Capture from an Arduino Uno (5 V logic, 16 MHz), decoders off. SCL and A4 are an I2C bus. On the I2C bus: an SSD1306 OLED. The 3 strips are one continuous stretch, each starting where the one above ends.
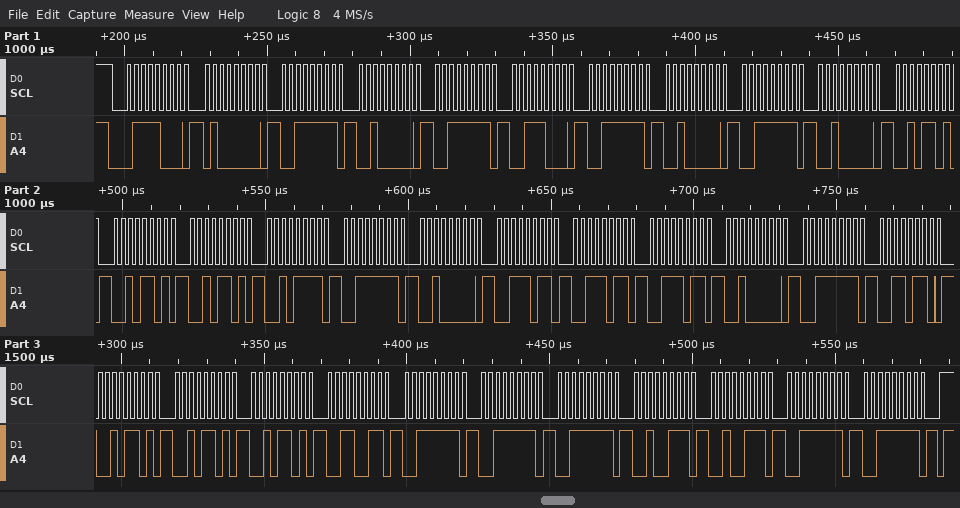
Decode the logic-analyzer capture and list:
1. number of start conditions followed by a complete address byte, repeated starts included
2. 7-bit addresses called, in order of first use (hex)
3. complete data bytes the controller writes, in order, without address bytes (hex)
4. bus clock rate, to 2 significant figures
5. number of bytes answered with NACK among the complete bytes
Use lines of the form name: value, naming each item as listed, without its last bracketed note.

number of start conditions followed by a complete address byte, repeated starts included: 1
7-bit addresses called, in order of first use: 0x3C
complete data bytes the controller writes, in order, without address bytes: 40 3F 20 3F 38 3F 20 3F 20 2D 2D 2D 2F 3F 20 3B 3B 3B 20 3F 36 2D 2D 2D 33 3F 3F 3F 27 27 3F 3F
bus clock rate, to 2 significant figures: 400 kHz
number of bytes answered with NACK among the complete bytes: 0
